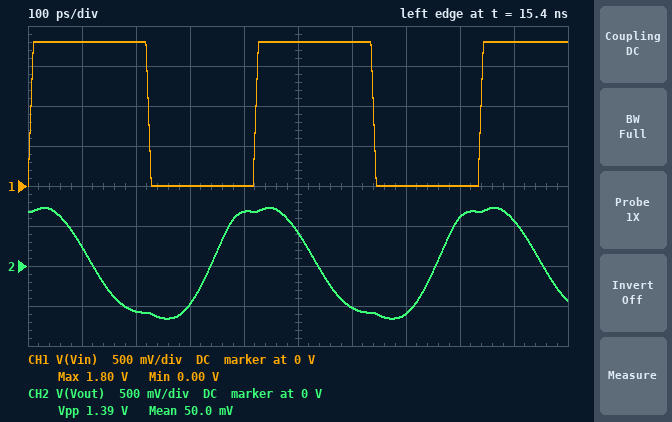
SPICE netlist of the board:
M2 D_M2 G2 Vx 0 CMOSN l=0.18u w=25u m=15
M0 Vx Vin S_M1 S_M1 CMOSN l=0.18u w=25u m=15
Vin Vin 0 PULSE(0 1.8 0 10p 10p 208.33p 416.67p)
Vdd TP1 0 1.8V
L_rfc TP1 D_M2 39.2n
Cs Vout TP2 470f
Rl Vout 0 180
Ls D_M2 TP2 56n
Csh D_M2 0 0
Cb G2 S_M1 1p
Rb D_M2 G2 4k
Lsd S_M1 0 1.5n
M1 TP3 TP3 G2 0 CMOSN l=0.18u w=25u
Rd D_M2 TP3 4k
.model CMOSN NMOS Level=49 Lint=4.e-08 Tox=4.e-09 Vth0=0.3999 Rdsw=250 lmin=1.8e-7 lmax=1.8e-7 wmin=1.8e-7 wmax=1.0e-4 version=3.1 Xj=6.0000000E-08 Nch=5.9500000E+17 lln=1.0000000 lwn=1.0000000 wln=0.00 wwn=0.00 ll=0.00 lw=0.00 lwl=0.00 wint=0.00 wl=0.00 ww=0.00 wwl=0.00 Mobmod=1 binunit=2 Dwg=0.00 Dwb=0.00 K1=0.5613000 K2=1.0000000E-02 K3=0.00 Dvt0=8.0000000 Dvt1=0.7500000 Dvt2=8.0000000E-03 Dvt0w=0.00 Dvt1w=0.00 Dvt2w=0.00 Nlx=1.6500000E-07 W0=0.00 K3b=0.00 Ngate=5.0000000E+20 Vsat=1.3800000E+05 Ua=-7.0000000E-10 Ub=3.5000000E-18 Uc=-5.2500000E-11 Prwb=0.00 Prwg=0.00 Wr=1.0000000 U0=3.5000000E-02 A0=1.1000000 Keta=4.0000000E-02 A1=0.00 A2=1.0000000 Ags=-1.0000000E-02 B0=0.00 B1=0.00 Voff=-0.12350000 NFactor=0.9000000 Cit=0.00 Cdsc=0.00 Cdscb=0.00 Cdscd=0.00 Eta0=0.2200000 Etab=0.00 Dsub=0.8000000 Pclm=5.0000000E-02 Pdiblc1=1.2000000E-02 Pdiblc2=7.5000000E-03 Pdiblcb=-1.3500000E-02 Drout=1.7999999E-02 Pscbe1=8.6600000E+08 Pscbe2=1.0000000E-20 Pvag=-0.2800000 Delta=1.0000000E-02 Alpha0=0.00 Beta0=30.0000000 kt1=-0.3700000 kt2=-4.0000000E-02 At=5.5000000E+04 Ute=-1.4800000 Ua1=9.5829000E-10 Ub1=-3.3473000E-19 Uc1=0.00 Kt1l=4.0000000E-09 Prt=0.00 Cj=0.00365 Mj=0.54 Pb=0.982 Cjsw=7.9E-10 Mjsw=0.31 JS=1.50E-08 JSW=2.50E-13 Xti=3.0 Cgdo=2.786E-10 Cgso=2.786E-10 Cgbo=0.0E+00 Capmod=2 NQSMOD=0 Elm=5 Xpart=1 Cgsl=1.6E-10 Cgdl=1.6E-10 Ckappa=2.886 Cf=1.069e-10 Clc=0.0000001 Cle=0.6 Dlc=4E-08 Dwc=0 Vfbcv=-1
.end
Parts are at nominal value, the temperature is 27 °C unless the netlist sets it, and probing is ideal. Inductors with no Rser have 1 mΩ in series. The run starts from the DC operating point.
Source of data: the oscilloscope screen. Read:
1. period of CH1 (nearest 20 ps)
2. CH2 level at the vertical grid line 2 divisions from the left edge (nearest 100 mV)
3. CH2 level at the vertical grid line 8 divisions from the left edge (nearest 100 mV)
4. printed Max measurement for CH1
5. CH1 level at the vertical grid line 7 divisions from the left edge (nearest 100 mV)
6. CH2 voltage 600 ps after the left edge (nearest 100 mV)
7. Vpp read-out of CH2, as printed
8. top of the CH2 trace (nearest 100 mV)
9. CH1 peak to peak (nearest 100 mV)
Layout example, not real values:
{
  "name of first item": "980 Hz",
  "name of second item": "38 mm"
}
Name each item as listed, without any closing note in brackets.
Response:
{
  "period of CH1": "420 ps",
  "CH2 level at the vertical grid line 2 divisions from the left edge": "-600 mV",
  "CH2 level at the vertical grid line 8 divisions from the left edge": "600 mV",
  "printed Max measurement for CH1": "1.80 V",
  "CH1 level at the vertical grid line 7 divisions from the left edge": "0 V",
  "CH2 voltage 600 ps after the left edge": "-500 mV",
  "Vpp read-out of CH2, as printed": "1.39 V",
  "top of the CH2 trace": "700 mV",
  "CH1 peak to peak": "1.8 V"
}
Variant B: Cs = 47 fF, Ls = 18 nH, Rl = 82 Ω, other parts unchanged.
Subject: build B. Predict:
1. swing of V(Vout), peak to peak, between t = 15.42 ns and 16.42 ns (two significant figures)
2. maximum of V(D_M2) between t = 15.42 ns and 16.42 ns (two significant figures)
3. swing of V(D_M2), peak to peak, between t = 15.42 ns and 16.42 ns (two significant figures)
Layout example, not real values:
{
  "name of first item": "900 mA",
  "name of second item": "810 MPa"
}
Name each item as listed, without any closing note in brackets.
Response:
{
  "swing of V(Vout), peak to peak, between t = 15.42 ns and 16.42 ns": "1.3 V",
  "maximum of V(D_M2) between t = 15.42 ns and 16.42 ns": "6.7 V",
  "swing of V(D_M2), peak to peak, between t = 15.42 ns and 16.42 ns": "8.1 V"
}
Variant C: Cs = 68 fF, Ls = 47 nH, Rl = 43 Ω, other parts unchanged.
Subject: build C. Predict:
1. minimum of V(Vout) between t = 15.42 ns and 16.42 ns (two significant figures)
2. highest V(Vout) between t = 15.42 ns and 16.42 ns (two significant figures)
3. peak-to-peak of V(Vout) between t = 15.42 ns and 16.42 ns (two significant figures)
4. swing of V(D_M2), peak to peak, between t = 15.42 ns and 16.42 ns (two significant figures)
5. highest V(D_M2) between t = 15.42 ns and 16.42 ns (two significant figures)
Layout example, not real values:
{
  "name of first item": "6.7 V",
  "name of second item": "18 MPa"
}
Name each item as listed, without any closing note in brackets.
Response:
{
  "minimum of V(Vout) between t = 15.42 ns and 16.42 ns": "-590 mV",
  "highest V(Vout) between t = 15.42 ns and 16.42 ns": "580 mV",
  "peak-to-peak of V(Vout) between t = 15.42 ns and 16.42 ns": "1.2 V",
  "swing of V(D_M2), peak to peak, between t = 15.42 ns and 16.42 ns": "12 V",
  "highest V(D_M2) between t = 15.42 ns and 16.42 ns": "10 V"
}
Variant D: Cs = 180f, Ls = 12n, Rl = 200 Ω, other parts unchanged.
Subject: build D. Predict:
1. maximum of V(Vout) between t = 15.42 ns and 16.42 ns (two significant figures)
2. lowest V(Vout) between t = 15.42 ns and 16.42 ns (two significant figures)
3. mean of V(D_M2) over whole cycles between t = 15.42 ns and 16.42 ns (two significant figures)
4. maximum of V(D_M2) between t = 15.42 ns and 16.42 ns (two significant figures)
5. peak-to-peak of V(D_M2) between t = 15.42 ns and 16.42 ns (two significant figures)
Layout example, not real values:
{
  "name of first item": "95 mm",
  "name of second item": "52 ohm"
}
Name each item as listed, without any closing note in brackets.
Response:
{
  "maximum of V(Vout) between t = 15.42 ns and 16.42 ns": "2.5 V",
  "lowest V(Vout) between t = 15.42 ns and 16.42 ns": "-2.7 V",
  "mean of V(D_M2) over whole cycles between t = 15.42 ns and 16.42 ns": "1.8 V",
  "maximum of V(D_M2) between t = 15.42 ns and 16.42 ns": "6.9 V",
  "peak-to-peak of V(D_M2) between t = 15.42 ns and 16.42 ns": "7.9 V"
}
